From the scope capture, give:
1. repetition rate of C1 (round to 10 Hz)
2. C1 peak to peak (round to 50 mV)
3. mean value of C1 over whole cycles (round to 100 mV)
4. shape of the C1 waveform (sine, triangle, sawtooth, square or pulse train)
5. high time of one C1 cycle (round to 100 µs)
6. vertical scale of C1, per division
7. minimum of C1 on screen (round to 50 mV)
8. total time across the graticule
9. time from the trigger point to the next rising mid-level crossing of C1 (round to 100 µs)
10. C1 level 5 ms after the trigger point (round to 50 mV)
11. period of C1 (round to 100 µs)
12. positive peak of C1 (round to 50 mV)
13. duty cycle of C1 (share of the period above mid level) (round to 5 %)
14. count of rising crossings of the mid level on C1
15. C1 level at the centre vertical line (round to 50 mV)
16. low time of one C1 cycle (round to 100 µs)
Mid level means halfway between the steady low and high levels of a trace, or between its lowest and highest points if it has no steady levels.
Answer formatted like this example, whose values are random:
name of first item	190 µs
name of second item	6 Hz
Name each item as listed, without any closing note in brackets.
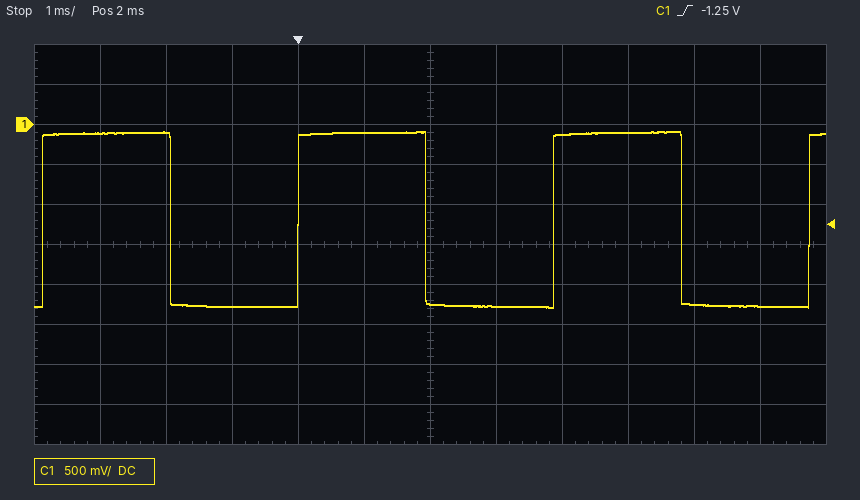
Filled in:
repetition rate of C1	260 Hz
C1 peak to peak	2.20 V
mean value of C1 over whole cycles	-1.2 V
shape of the C1 waveform	square
high time of one C1 cycle	1.9 ms
vertical scale of C1, per division	500 mV
minimum of C1 on screen	-2.30 V
total time across the graticule	12 ms
time from the trigger point to the next rising mid-level crossing of C1	3.9 ms
C1 level 5 ms after the trigger point	-100 mV
period of C1	3.9 ms
positive peak of C1	-100 mV
duty cycle of C1 (share of the period above mid level)	50 %
count of rising crossings of the mid level on C1	4
C1 level at the centre vertical line	-2.25 V
low time of one C1 cycle	1.9 ms
